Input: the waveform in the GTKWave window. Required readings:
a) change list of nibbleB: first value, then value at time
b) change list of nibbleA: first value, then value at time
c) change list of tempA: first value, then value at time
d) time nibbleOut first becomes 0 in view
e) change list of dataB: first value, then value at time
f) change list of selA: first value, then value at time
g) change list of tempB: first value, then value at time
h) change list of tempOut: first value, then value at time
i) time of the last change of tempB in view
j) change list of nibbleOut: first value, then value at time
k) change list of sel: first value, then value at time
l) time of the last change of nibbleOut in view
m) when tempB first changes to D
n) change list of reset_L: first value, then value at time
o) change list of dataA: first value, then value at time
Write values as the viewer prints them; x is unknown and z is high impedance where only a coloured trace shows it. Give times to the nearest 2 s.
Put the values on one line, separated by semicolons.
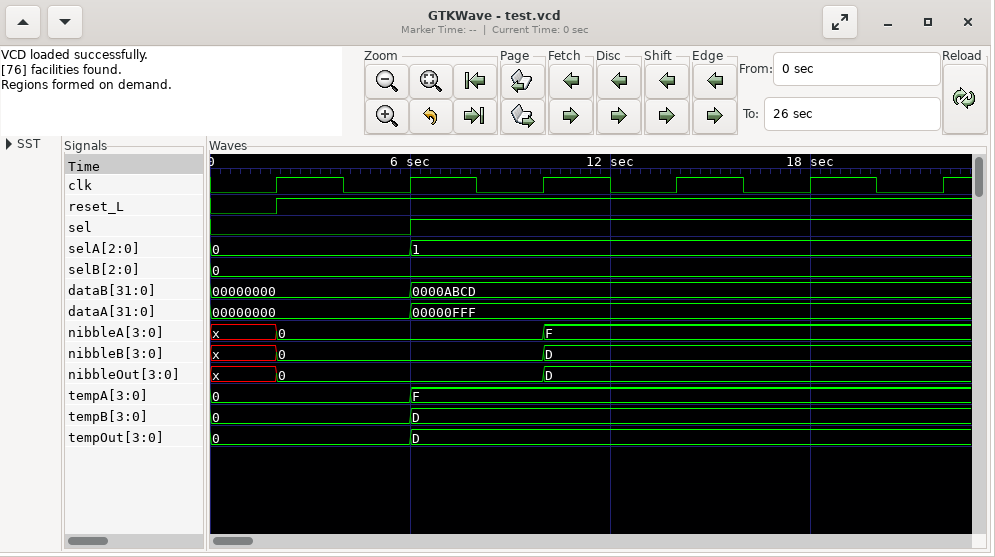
x, 0 at 2 s, D at 10 s; x, 0 at 2 s, F at 10 s; 0, F at 6 s; 2 s; 00000000, 0000ABCD at 6 s; 0, 1 at 6 s; 0, D at 6 s; 0, D at 6 s; 6 s; x, 0 at 2 s, D at 10 s; 0, 1 at 6 s; 10 s; 6 s; 0, 1 at 2 s; 00000000, 00000FFF at 6 s
